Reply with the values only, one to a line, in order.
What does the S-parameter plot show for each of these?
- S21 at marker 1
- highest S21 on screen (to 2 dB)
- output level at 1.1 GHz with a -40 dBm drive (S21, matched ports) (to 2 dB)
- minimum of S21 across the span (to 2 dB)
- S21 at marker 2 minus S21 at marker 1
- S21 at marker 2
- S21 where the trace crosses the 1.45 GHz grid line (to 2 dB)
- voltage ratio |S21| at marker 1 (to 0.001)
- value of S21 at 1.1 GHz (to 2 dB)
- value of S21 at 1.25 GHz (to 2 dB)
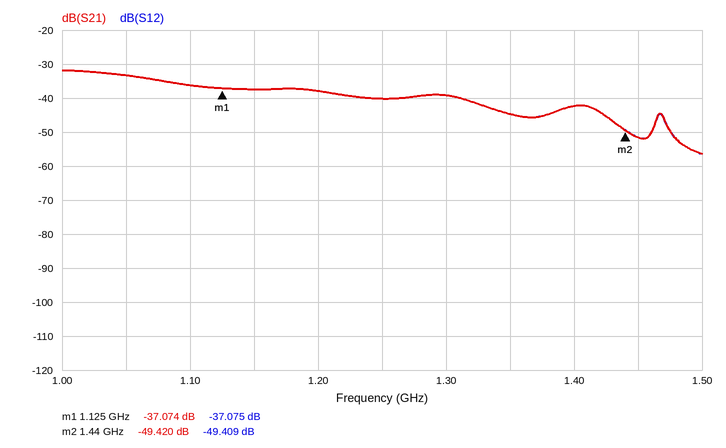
-37.074 dB
-32 dB
-76 dBm
-56 dB
-12.346 dB
-49.420 dB
-52 dB
0.014
-36 dB
-40 dB
